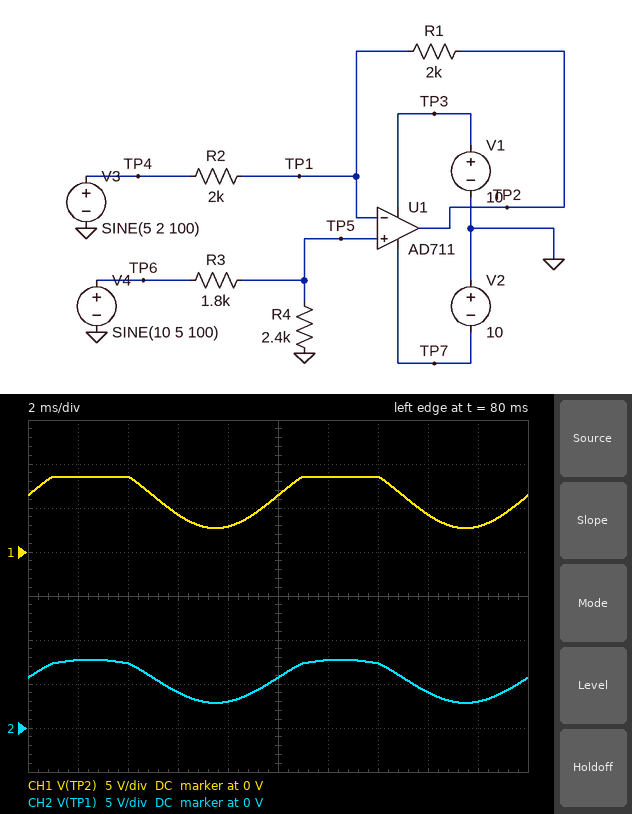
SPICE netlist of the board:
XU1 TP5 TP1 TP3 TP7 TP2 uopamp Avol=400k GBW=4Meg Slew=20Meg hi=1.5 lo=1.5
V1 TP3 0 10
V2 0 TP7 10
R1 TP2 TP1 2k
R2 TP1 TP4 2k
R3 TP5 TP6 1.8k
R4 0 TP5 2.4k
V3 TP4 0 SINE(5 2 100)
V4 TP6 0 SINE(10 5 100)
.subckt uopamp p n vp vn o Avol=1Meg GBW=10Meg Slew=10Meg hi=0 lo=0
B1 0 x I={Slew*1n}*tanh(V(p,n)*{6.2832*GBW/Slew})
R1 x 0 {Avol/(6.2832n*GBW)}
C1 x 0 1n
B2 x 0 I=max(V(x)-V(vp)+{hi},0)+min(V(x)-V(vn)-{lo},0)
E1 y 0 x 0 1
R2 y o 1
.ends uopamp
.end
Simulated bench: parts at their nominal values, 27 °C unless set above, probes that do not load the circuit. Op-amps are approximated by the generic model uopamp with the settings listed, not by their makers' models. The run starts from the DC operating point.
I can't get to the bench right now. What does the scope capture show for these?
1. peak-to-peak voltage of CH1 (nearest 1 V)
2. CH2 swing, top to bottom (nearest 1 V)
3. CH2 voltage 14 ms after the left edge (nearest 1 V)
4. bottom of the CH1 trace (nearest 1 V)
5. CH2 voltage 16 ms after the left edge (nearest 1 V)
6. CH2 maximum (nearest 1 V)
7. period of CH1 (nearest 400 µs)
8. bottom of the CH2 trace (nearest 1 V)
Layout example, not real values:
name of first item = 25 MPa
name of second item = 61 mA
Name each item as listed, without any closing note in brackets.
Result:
peak-to-peak voltage of CH1 = 6 V
CH2 swing, top to bottom = 5 V
CH2 voltage 14 ms after the left edge = 7 V
bottom of the CH1 trace = 3 V
CH2 voltage 16 ms after the left edge = 4 V
CH2 maximum = 8 V
period of CH1 = 10.0 ms
bottom of the CH2 trace = 3 V
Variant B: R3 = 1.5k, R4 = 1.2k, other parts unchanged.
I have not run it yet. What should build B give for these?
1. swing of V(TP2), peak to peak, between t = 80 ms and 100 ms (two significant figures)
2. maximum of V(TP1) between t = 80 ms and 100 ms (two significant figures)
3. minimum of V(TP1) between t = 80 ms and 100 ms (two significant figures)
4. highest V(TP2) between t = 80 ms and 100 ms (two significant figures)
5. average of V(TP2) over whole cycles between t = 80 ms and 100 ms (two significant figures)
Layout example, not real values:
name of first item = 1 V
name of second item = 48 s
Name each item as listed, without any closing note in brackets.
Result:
swing of V(TP2), peak to peak, between t = 80 ms and 100 ms = 4.9 V
maximum of V(TP1) between t = 80 ms and 100 ms = 6.7 V
minimum of V(TP1) between t = 80 ms and 100 ms = 2.2 V
highest V(TP2) between t = 80 ms and 100 ms = 6.3 V
average of V(TP2) over whole cycles between t = 80 ms and 100 ms = 3.9 V
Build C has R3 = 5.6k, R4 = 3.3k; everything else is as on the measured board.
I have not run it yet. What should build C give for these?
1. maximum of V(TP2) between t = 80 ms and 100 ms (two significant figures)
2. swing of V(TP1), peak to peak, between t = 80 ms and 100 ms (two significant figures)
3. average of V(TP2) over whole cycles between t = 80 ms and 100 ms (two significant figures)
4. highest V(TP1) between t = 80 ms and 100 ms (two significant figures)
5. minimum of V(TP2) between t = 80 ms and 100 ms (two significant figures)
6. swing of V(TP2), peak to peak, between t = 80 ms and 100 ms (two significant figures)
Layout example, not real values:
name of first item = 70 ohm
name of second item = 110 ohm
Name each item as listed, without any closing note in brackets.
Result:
maximum of V(TP2) between t = 80 ms and 100 ms = 4.1 V
swing of V(TP1), peak to peak, between t = 80 ms and 100 ms = 3.7 V
average of V(TP2) over whole cycles between t = 80 ms and 100 ms = 2.4 V
highest V(TP1) between t = 80 ms and 100 ms = 5.6 V
minimum of V(TP2) between t = 80 ms and 100 ms = 710 mV
swing of V(TP2), peak to peak, between t = 80 ms and 100 ms = 3.4 V
